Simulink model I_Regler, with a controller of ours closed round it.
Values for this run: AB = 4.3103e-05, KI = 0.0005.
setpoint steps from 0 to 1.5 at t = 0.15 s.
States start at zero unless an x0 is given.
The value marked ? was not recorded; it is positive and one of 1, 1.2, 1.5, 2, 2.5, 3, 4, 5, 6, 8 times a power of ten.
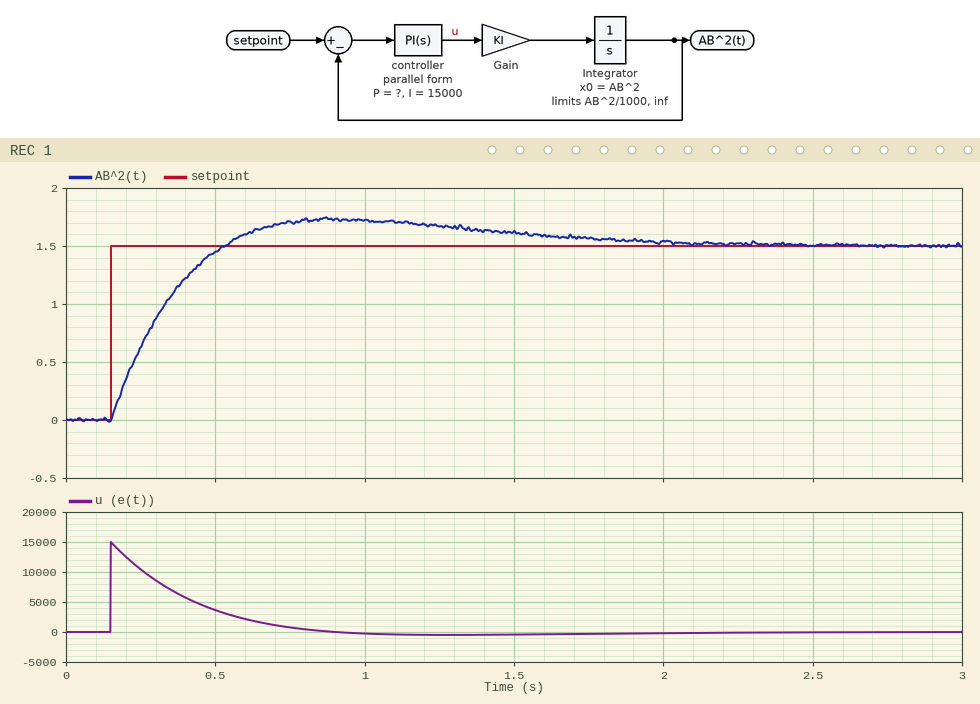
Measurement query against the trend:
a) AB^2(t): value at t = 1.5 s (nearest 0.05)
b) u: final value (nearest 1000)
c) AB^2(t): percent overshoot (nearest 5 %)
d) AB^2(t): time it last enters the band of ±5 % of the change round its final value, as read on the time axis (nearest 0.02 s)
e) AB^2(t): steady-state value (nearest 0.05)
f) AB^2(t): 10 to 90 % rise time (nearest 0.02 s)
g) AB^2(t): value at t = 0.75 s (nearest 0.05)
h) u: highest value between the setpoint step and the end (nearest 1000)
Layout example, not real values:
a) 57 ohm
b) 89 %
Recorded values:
a) 1.60
b) 0
c) 15 %
d) 1.70 s
e) 1.50
f) 0.28 s
g) 1.70
h) 15000
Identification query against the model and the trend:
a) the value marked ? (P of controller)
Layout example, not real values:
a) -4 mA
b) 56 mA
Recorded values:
a) 10000
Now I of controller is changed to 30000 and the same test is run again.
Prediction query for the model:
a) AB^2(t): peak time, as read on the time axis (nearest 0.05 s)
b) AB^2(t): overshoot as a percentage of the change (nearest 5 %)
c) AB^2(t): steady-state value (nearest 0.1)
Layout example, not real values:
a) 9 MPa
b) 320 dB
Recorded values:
a) 0.75 s
b) 25 %
c) 1.5
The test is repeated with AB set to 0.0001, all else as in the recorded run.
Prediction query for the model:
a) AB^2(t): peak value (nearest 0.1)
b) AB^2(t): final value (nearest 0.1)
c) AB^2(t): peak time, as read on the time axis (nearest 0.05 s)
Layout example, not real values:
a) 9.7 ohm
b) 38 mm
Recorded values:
a) 1.7
b) 1.5
c) 0.90 s
